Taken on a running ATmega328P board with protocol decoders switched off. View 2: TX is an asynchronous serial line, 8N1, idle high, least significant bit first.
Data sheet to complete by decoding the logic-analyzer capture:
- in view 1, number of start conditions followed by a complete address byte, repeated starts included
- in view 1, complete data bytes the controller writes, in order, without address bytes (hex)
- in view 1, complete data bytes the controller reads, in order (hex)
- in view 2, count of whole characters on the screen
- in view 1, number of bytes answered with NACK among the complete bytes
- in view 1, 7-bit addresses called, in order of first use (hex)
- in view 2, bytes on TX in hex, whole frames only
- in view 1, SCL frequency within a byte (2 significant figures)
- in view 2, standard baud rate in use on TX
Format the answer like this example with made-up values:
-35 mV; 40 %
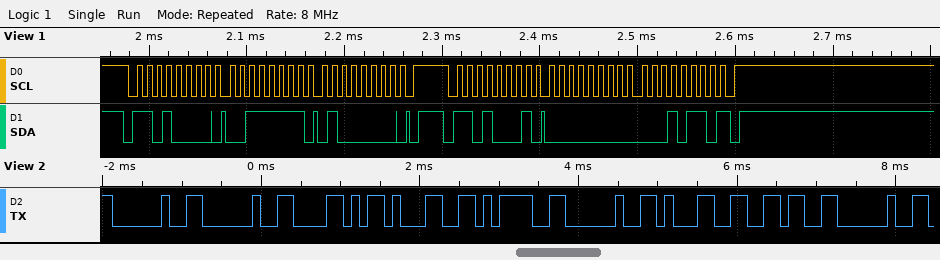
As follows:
2; 3F 40; 00 16; 9; 1; 0x68; 20 20 58 31 3D 20 31 36 20; 100 kHz; 9600 baud
